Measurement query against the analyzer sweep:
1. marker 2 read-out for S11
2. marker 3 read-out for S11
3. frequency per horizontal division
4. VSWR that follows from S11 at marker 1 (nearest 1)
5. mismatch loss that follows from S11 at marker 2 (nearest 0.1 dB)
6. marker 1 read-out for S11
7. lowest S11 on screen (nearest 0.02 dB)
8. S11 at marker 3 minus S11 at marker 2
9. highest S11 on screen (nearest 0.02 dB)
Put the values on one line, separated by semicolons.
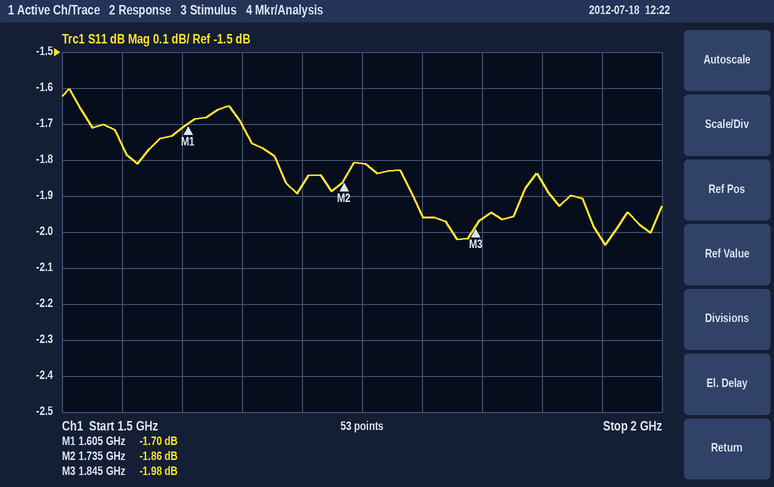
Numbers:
-1.86 dB; -1.98 dB; 50 MHz; 10; 4.6 dB; -1.70 dB; -2.04 dB; -0.12 dB; -1.60 dB
